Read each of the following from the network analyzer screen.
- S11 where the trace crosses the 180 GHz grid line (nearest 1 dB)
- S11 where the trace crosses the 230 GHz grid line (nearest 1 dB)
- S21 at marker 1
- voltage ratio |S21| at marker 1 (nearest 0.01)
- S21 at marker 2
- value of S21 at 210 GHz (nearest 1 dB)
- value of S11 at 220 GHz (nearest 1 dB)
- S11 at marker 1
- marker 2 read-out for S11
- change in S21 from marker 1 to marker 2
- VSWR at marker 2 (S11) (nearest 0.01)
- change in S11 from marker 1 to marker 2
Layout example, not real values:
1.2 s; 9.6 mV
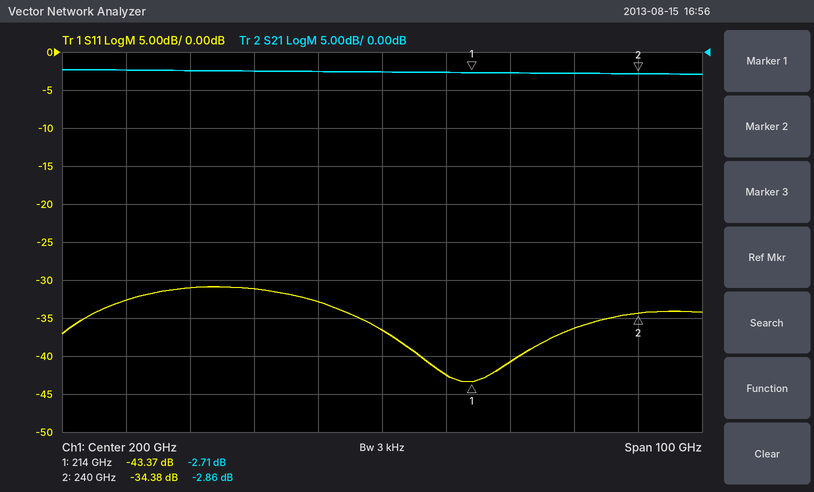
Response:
-31 dB; -36 dB; -2.71 dB; 0.73; -2.86 dB; -3 dB; -41 dB; -43.37 dB; -34.38 dB; -0.15 dB; 1.04; 8.99 dB
